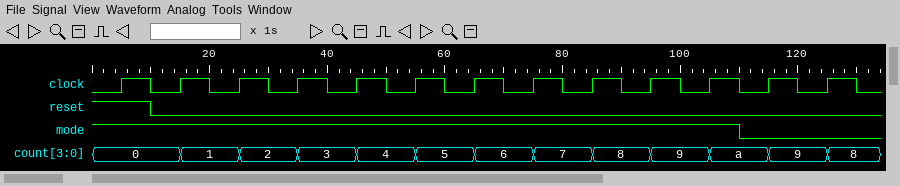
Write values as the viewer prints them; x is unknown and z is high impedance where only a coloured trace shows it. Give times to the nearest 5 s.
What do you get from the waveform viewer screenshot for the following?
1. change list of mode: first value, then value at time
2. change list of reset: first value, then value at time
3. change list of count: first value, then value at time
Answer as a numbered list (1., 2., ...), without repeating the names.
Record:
1. 1, 0 at 110 s
2. 1, 0 at 10 s
3. 0, 1 at 15 s, 2 at 25 s, 3 at 35 s, 4 at 45 s, 5 at 55 s, 6 at 65 s, 7 at 75 s, 8 at 85 s, 9 at 95 s, a at 105 s, 9 at 115 s, 8 at 125 s
